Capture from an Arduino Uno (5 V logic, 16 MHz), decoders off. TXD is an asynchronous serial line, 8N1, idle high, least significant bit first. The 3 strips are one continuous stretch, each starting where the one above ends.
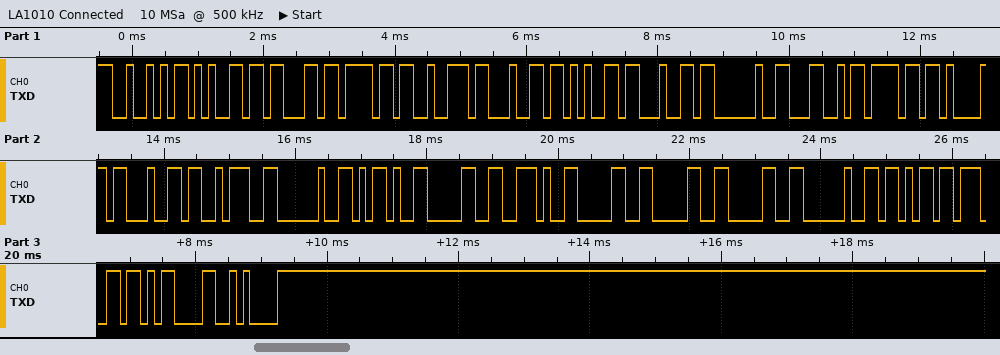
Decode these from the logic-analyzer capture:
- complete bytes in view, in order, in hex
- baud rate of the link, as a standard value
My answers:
52 65 63 6F 72 64 65 64 20 4C 6F 61 64 3A 20 2D 30 2E 30 30 30 20 6B 67 0D 0A
9600 baud
